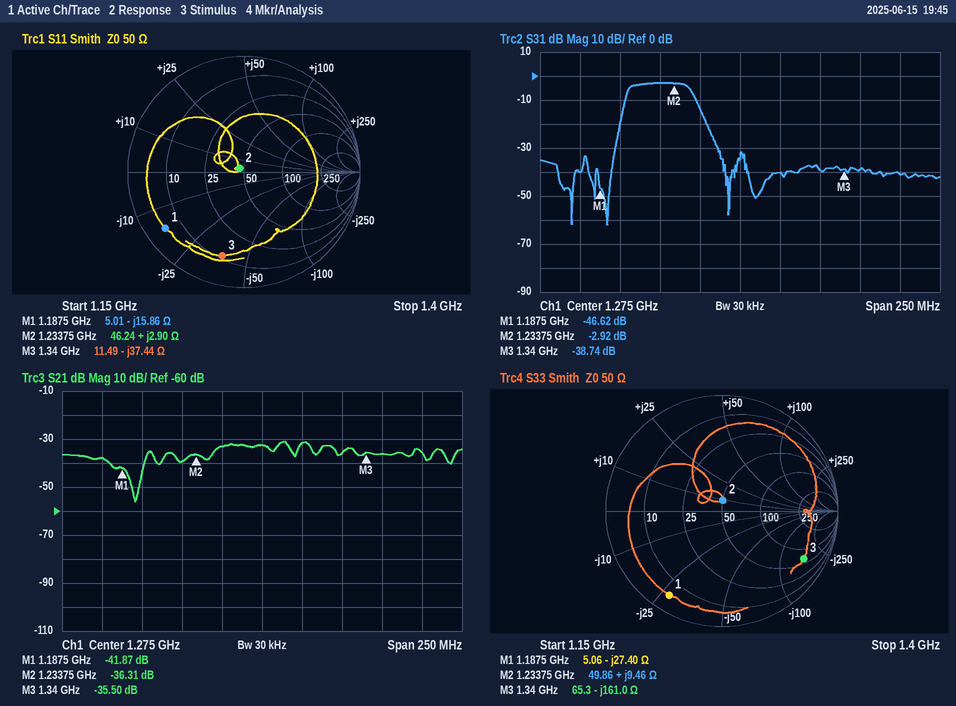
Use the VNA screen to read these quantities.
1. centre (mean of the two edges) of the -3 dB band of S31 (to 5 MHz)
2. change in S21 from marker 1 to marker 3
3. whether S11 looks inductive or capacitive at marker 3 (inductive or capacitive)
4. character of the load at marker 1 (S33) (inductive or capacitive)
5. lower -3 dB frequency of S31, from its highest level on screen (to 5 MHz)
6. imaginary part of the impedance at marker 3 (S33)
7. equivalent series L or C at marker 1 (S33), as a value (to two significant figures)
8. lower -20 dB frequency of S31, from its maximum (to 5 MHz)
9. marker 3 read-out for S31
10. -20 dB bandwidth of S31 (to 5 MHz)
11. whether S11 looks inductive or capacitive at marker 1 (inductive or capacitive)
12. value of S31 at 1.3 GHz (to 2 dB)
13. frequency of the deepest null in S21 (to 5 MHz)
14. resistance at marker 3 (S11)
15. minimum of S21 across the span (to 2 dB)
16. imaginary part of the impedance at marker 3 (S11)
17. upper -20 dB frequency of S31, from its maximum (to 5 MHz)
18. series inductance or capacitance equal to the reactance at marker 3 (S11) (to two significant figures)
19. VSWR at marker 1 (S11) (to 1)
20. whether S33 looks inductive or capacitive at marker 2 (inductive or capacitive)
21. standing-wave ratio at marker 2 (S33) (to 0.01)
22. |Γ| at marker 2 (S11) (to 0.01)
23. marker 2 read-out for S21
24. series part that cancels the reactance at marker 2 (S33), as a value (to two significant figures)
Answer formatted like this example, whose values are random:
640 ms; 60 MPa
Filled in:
1.225 GHz; 6.37 dB; capacitive; capacitive; 1.205 GHz; -161.0 Ω; 4.9 pF; 1.200 GHz; -38.74 dB; 55 MHz; capacitive; -40 dB; 1.195 GHz; 11.49 Ω; -56 dB; -37.44 Ω; 1.255 GHz; 3.2 pF; 11; inductive; 1.21; 0.05; -36.31 dB; 14 pF
